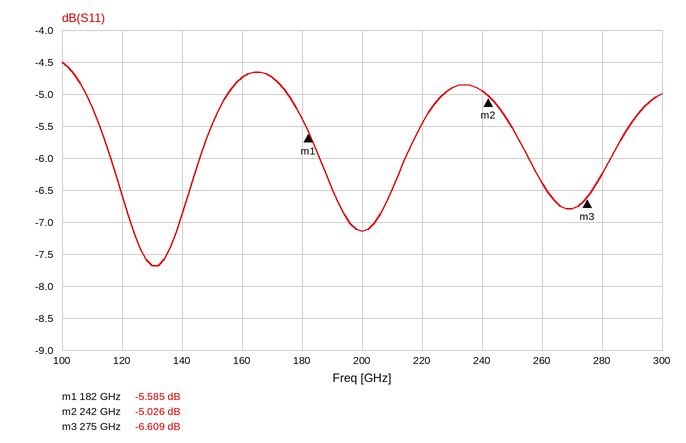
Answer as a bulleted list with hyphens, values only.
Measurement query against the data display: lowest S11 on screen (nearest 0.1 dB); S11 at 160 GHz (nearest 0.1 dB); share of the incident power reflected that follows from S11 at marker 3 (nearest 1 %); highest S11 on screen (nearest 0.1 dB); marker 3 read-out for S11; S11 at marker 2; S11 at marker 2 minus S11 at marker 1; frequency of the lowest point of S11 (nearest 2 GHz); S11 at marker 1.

- -7.7 dB
- -4.7 dB
- 22 %
- -4.5 dB
- -6.609 dB
- -5.026 dB
- 0.559 dB
- 130 GHz
- -5.585 dB
